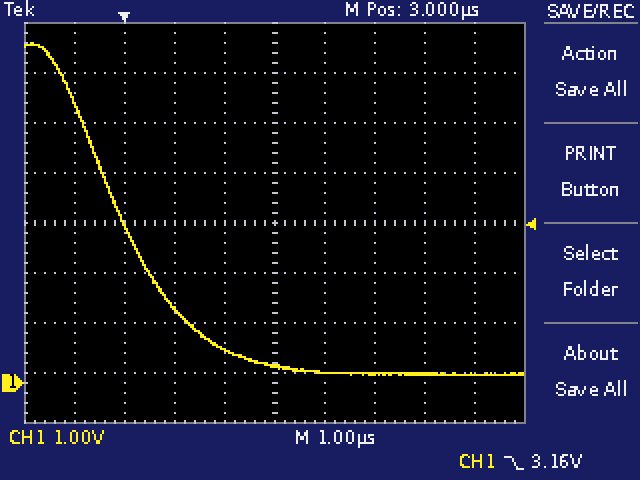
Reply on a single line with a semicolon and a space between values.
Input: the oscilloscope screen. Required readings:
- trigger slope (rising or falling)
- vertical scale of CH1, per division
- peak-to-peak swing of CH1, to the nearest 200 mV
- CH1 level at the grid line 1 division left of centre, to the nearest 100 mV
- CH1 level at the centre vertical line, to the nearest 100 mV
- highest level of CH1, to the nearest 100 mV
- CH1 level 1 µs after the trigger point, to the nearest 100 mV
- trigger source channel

falling; 1 V; 6.6 V; 700 mV; 300 mV; 6.8 V; 1.5 V; CH1
